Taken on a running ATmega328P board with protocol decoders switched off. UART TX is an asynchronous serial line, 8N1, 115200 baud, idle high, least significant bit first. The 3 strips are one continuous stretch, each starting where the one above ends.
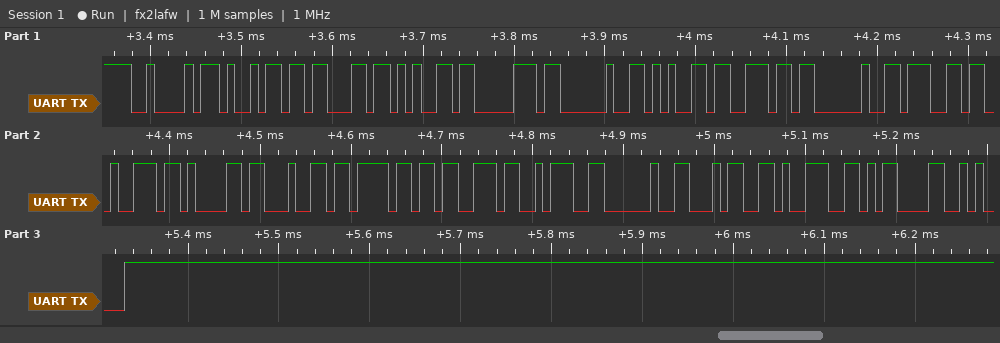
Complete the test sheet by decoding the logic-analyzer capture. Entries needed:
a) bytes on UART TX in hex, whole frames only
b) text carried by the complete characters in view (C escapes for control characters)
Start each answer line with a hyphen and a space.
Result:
- 0x42 0x69 0x63 0x65 0x70 0x20 0x65 0x6E 0x20 0x67 0x72 0x61 0x64 0x6F 0x73 0x3A 0x20 0x34 0x39 0x0D 0x0A
- "Bicep en grados: 49\r\n"
